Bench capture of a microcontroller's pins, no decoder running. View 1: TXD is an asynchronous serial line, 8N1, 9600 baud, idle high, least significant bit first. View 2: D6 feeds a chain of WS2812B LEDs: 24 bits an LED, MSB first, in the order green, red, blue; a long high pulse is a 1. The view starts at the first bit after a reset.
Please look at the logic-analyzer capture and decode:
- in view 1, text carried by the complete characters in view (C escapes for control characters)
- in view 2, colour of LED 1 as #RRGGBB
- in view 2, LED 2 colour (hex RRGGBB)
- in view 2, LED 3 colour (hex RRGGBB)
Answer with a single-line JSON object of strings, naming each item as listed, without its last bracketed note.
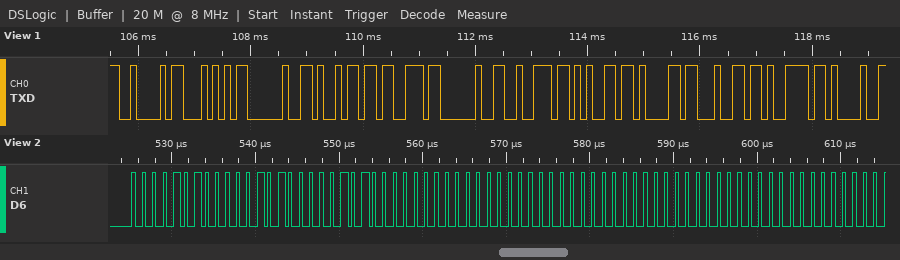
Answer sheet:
{"in view 1, text carried by the complete characters in view": "\"BT is ready!\"", "in view 2, colour of LED 1 as #RRGGBB": "#0A0A0A", "in view 2, LED 2 colour": "#000000", "in view 2, LED 3 colour": "#000000"}
